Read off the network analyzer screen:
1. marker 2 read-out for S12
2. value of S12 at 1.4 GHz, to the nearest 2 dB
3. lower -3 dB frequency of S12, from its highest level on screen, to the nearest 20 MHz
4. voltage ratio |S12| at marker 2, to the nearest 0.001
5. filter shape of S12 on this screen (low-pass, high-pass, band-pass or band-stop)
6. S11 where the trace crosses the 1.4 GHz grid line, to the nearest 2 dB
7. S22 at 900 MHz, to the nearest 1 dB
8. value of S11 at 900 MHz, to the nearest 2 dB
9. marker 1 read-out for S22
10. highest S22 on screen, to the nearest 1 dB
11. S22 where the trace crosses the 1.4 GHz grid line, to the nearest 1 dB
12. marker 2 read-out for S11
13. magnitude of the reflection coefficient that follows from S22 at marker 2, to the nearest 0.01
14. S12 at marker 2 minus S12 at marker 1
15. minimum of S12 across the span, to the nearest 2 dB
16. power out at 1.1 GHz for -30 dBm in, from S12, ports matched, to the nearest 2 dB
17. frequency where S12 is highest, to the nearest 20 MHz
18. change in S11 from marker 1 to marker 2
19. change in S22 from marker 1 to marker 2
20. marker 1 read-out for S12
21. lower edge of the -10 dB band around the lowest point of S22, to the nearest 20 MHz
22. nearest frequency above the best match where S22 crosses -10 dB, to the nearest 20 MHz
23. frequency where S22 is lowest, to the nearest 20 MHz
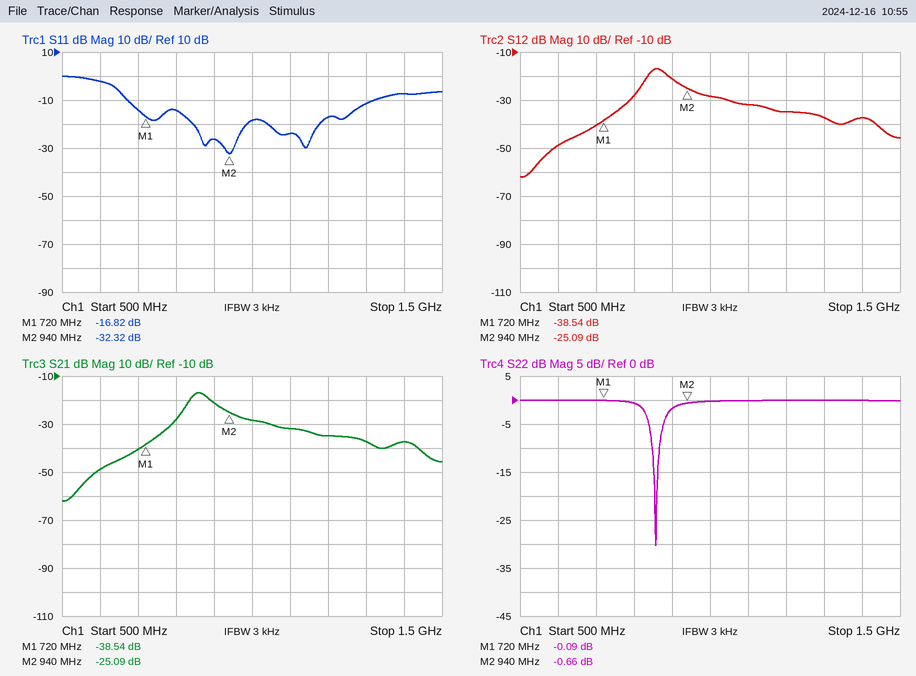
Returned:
-25.09 dB
-38 dB
840 MHz
0.056
band-pass
-8 dB
-2 dB
-26 dB
-0.09 dB
0 dB
0 dB
-32.32 dB
0.93
13.45 dB
-62 dB
-62 dBm
860 MHz
-15.50 dB
-0.57 dB
-38.54 dB
840 MHz
860 MHz
860 MHz
